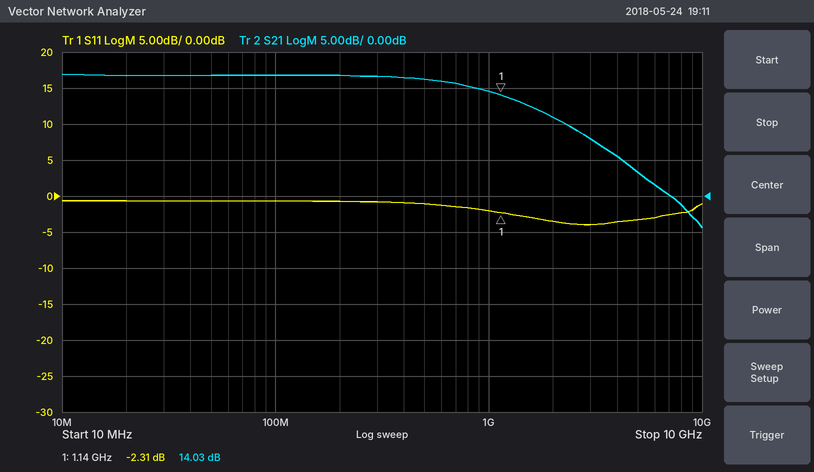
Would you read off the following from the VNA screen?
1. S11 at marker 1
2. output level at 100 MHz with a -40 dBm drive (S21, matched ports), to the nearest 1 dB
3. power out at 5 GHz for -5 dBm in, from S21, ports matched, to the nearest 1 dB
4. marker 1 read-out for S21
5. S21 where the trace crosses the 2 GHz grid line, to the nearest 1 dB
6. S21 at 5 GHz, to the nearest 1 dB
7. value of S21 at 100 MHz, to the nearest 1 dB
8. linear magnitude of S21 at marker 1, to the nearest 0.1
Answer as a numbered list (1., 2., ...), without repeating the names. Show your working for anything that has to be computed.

1. -2.31 dB
2. -40 dBm + (17 dB) = -23 dBm
3. -5 dBm + (3 dB) = -2 dBm
4. 14.03 dB
5. 11 dB
6. 3 dB
7. 17 dB
8. 10^(14.03/20) ≈ 5.0
